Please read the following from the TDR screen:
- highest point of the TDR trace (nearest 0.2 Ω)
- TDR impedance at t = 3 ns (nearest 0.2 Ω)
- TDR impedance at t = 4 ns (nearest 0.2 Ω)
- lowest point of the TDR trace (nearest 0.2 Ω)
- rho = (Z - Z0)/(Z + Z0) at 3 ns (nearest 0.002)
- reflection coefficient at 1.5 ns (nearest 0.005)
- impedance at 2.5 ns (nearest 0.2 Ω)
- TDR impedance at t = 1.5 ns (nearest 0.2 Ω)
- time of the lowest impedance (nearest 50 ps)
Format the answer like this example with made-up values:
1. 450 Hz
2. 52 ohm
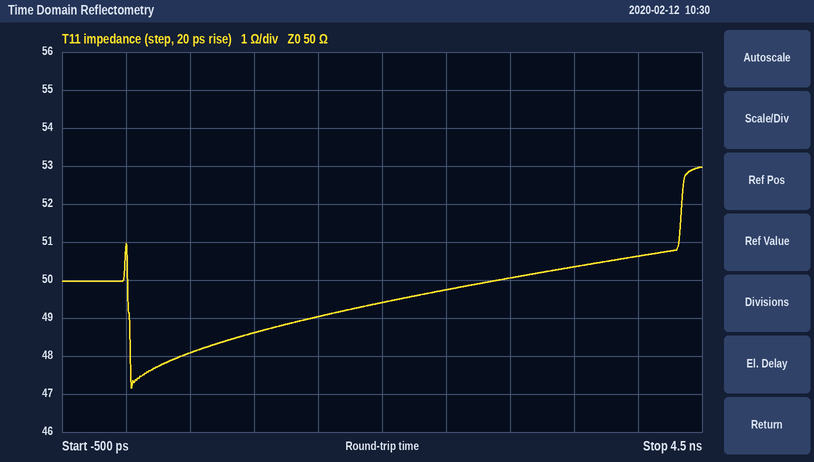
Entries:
1. 53.0 Ω
2. 50.0 Ω
3. 50.6 Ω
4. 47.2 Ω
5. 0.000
6. -0.010
7. 49.8 Ω
8. 49.0 Ω
9. 50 ps
